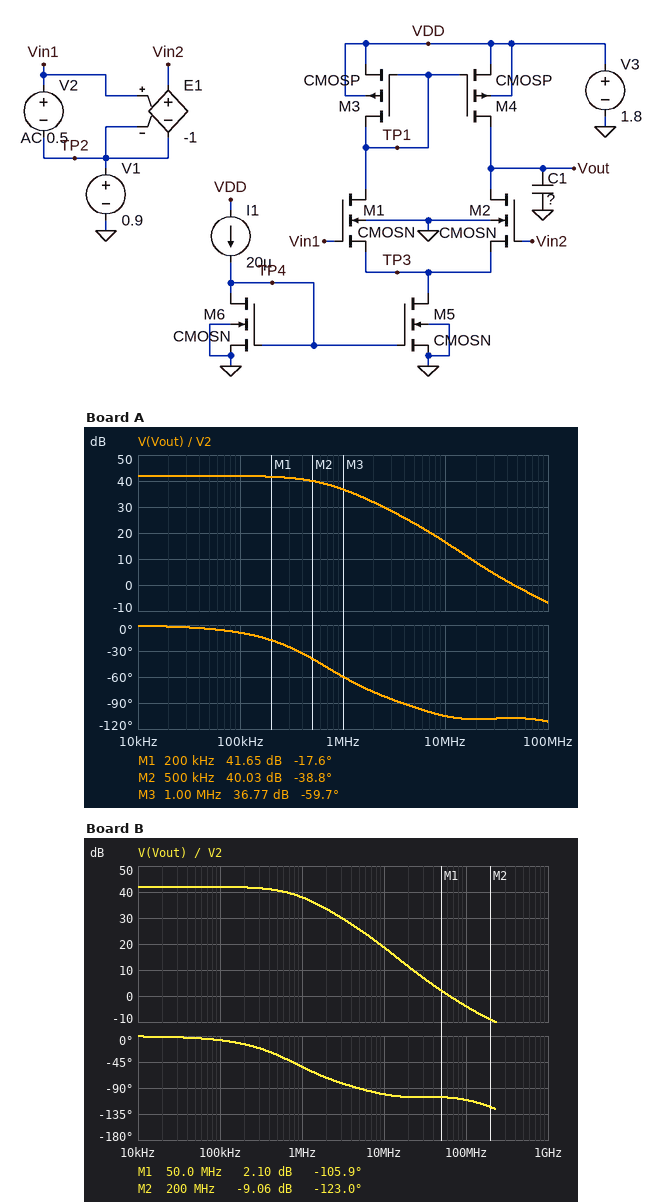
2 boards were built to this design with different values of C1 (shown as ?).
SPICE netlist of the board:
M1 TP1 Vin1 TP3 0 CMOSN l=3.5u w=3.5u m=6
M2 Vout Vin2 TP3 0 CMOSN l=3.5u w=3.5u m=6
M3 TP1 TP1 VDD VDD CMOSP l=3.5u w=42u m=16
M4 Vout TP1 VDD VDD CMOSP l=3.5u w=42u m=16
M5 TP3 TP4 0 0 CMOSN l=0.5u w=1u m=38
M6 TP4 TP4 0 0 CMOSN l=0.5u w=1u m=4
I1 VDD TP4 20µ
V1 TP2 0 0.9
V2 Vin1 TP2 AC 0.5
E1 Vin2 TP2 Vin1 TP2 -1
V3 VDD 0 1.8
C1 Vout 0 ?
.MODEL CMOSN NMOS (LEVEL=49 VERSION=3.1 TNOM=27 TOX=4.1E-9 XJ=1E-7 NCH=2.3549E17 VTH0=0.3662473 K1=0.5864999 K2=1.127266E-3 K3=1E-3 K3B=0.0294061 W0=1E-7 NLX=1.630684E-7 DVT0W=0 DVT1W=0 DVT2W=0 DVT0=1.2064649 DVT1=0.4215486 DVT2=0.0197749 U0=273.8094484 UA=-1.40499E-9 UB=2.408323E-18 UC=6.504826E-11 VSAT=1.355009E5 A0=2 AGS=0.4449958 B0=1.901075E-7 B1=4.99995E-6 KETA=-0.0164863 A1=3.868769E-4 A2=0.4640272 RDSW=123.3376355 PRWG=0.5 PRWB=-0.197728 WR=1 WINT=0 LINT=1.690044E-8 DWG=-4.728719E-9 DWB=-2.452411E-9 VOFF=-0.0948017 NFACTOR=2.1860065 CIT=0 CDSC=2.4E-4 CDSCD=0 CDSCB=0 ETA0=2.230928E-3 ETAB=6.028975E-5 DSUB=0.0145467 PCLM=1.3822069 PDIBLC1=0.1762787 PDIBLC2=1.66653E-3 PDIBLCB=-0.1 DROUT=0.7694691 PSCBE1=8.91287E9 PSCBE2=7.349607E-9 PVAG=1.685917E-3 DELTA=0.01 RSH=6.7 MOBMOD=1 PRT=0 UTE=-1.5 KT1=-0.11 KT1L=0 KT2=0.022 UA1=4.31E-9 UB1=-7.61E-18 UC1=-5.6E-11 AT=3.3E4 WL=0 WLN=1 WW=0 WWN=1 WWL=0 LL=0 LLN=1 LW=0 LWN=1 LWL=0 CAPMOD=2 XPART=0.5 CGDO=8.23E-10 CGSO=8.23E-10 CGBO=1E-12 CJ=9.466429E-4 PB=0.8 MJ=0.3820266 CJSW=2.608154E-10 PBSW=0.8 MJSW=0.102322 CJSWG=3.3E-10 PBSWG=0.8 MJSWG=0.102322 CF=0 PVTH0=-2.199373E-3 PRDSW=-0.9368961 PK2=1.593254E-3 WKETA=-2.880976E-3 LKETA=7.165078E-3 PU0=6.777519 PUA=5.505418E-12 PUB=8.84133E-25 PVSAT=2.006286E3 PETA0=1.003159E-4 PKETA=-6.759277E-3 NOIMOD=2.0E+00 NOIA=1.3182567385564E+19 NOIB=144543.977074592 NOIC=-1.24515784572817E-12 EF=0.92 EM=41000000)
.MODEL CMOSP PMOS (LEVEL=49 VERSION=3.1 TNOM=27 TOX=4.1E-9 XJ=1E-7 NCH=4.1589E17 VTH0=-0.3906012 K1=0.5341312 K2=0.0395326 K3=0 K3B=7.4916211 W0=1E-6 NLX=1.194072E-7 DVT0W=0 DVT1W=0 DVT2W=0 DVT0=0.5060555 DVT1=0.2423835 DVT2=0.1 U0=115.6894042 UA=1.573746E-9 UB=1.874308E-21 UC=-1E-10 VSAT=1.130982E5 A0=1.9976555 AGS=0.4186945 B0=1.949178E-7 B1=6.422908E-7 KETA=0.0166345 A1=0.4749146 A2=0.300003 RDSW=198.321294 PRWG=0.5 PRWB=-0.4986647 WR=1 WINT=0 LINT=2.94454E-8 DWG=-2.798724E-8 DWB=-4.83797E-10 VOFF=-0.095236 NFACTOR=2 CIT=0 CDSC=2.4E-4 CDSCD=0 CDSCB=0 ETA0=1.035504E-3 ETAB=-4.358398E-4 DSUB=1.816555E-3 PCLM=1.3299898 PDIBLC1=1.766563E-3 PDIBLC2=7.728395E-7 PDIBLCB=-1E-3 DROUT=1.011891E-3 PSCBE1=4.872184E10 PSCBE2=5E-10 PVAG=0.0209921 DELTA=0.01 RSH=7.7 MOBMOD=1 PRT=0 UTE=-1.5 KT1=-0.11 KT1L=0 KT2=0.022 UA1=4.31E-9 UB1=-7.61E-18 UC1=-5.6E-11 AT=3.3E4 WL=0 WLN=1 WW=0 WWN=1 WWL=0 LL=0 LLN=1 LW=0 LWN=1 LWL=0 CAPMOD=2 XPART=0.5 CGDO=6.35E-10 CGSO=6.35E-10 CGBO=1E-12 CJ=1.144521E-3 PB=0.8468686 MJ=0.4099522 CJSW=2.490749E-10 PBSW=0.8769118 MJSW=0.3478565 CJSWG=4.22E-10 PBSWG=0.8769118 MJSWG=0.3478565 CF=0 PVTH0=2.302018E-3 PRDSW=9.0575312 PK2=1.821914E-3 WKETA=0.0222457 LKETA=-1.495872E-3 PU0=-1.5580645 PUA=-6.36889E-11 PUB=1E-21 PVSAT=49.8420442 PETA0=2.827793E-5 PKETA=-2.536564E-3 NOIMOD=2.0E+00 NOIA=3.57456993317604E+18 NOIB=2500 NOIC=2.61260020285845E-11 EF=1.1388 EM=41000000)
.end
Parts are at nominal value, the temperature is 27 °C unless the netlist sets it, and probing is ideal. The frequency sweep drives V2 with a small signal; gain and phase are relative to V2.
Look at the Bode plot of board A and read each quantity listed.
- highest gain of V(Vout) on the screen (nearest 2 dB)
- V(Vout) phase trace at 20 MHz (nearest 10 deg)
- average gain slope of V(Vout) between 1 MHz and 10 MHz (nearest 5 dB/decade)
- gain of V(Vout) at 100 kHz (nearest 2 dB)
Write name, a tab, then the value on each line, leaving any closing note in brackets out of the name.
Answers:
highest gain of V(Vout) on the screen	42 dB
V(Vout) phase trace at 20 MHz	-110 deg
average gain slope of V(Vout) between 1 MHz and 10 MHz	-20 dB/decade
gain of V(Vout) at 100 kHz	42 dB
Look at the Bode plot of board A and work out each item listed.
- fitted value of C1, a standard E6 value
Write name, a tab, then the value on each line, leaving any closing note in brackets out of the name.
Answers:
fitted value of C1, a standard E6 value	680 fF
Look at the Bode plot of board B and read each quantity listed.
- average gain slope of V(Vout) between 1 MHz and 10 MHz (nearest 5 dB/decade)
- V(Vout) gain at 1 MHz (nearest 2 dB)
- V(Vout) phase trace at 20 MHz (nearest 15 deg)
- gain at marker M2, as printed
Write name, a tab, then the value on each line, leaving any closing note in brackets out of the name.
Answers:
average gain slope of V(Vout) between 1 MHz and 10 MHz	-20 dB/decade
V(Vout) gain at 1 MHz	38 dB
V(Vout) phase trace at 20 MHz	-105 deg
gain at marker M2, as printed	-9.06 dB
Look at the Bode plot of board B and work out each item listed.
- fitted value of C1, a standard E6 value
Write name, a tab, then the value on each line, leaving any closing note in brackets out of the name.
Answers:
fitted value of C1, a standard E6 value	330 fF
